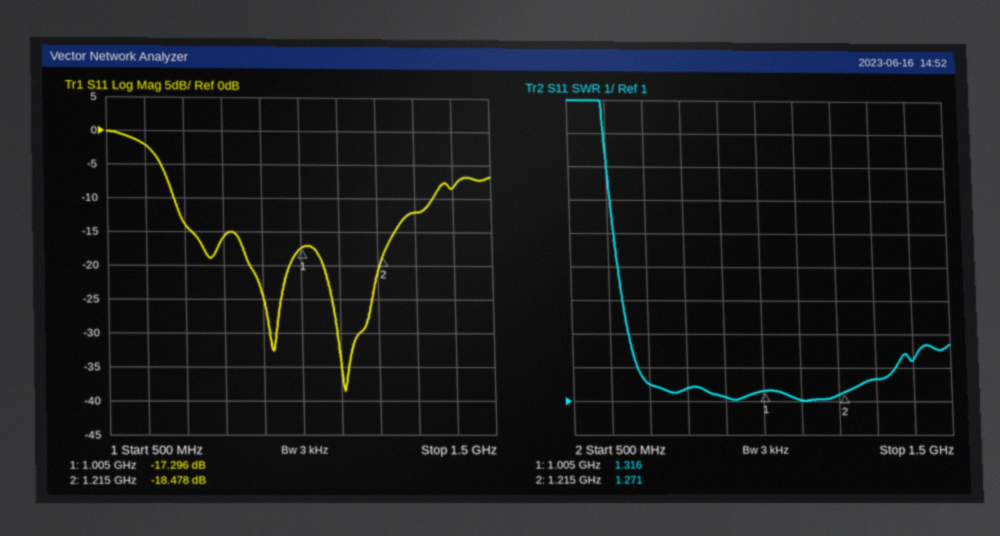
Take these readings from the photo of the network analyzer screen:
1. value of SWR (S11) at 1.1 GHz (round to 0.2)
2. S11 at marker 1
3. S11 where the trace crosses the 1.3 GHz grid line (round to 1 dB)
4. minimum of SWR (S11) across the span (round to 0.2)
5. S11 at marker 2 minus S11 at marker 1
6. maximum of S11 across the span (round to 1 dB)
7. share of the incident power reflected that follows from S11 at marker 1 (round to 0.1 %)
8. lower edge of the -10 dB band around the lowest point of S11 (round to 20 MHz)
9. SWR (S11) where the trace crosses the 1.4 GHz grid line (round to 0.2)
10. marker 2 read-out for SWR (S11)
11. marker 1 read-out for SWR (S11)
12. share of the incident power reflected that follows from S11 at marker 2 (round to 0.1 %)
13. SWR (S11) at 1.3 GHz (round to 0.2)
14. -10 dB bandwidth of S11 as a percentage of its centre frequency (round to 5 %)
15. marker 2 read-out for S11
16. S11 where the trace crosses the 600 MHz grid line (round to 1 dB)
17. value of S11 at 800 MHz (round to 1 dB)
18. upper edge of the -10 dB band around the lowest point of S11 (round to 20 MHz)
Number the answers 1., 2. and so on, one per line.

1. 1.0
2. -17.296 dB
3. -12 dB
4. 1.0
5. -1.182 dB
6. 0 dB
7. 1.9 %
8. 680 MHz
9. 2.2
10. 1.271
11. 1.316
12. 1.4 %
13. 1.6
14. 65 %
15. -18.478 dB
16. -2 dB
17. -16 dB
18. 1.34 GHz
